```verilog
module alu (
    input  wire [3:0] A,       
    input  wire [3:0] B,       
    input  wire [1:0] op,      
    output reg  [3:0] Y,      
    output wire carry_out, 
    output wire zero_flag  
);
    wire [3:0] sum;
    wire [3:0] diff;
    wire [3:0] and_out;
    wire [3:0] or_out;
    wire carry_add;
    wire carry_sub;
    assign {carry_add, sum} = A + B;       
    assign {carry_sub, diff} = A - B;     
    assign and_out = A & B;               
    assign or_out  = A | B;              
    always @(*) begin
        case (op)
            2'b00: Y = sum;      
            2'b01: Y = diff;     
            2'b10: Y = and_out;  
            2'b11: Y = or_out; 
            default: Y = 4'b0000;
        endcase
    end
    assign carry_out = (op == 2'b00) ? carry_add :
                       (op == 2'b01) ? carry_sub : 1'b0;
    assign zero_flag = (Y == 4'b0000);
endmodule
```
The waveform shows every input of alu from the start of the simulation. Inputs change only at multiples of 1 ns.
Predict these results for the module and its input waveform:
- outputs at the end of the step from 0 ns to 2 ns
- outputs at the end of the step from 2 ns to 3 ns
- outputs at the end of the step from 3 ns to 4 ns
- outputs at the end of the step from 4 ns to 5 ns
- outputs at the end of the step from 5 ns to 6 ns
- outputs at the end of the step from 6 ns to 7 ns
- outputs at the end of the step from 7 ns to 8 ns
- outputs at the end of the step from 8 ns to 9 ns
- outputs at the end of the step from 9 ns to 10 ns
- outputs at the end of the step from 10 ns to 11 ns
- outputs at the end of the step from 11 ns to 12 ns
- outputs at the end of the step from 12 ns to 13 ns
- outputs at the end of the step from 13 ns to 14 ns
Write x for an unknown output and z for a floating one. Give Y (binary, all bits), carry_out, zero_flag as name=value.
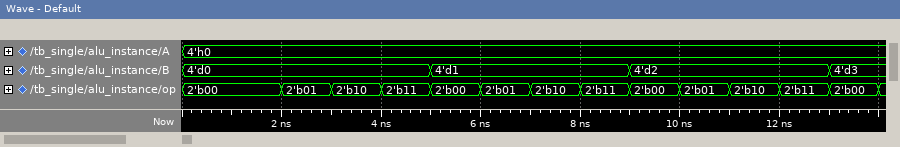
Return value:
Y=0000, carry_out=0, zero_flag=1
Y=0000, carry_out=0, zero_flag=1
Y=0000, carry_out=0, zero_flag=1
Y=0000, carry_out=0, zero_flag=1
Y=0001, carry_out=0, zero_flag=0
Y=1111, carry_out=1, zero_flag=0
Y=0000, carry_out=0, zero_flag=1
Y=0001, carry_out=0, zero_flag=0
Y=0010, carry_out=0, zero_flag=0
Y=1110, carry_out=1, zero_flag=0
Y=0000, carry_out=0, zero_flag=1
Y=0010, carry_out=0, zero_flag=0
Y=0011, carry_out=0, zero_flag=0
